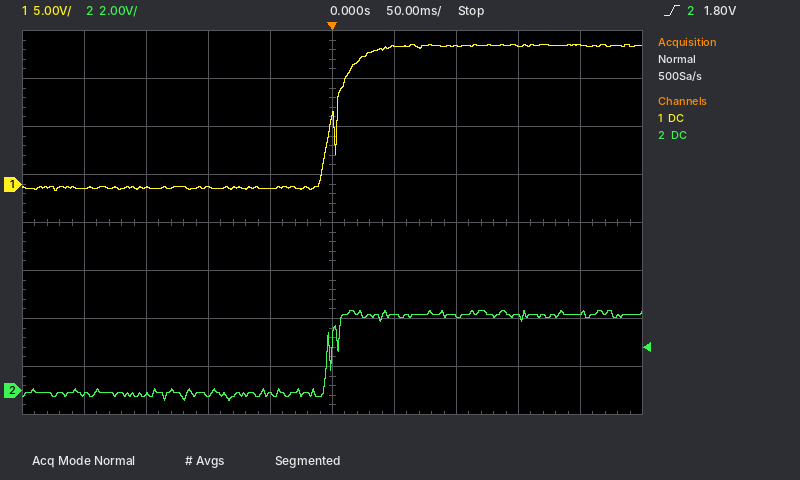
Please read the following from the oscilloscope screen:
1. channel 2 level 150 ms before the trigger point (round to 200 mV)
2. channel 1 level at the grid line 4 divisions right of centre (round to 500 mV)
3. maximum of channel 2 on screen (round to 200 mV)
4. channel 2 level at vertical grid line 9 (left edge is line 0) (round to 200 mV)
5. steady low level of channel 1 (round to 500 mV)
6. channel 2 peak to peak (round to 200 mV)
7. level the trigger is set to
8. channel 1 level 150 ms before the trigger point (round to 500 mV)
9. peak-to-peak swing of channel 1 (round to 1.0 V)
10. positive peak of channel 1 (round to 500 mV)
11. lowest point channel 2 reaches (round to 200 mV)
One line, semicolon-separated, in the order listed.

-200 mV; 14.5 V; 3.4 V; 3.2 V; -500 mV; 3.8 V; 1.80 V; -500 mV; 15.0 V; 14.5 V; -400 mV
